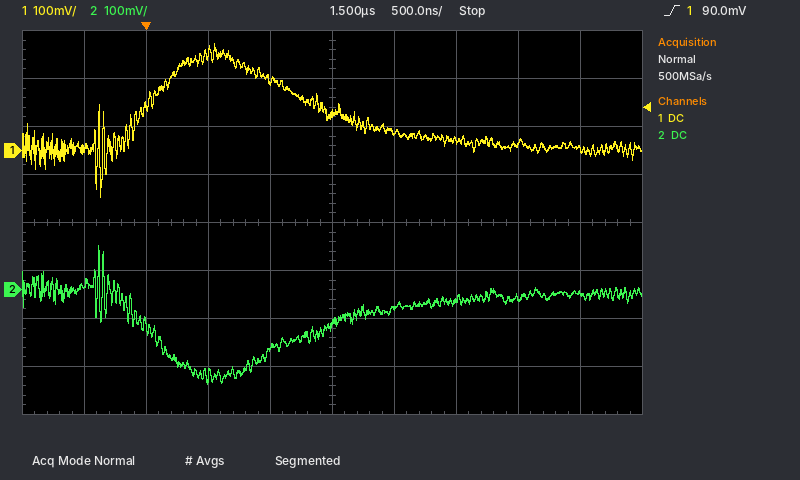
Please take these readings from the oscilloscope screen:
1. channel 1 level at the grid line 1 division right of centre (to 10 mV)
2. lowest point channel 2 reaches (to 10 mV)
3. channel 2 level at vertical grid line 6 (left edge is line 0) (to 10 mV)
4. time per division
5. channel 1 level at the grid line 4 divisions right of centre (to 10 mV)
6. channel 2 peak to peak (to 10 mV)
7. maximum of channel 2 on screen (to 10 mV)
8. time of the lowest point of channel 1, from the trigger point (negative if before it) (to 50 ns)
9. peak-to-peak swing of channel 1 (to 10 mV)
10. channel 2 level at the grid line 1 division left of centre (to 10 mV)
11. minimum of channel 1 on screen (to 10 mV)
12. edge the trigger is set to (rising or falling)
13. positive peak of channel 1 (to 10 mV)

40 mV
-200 mV
-40 mV
500 ns
0 mV
290 mV
90 mV
-350 ns
320 mV
-120 mV
-100 mV
rising
220 mV
